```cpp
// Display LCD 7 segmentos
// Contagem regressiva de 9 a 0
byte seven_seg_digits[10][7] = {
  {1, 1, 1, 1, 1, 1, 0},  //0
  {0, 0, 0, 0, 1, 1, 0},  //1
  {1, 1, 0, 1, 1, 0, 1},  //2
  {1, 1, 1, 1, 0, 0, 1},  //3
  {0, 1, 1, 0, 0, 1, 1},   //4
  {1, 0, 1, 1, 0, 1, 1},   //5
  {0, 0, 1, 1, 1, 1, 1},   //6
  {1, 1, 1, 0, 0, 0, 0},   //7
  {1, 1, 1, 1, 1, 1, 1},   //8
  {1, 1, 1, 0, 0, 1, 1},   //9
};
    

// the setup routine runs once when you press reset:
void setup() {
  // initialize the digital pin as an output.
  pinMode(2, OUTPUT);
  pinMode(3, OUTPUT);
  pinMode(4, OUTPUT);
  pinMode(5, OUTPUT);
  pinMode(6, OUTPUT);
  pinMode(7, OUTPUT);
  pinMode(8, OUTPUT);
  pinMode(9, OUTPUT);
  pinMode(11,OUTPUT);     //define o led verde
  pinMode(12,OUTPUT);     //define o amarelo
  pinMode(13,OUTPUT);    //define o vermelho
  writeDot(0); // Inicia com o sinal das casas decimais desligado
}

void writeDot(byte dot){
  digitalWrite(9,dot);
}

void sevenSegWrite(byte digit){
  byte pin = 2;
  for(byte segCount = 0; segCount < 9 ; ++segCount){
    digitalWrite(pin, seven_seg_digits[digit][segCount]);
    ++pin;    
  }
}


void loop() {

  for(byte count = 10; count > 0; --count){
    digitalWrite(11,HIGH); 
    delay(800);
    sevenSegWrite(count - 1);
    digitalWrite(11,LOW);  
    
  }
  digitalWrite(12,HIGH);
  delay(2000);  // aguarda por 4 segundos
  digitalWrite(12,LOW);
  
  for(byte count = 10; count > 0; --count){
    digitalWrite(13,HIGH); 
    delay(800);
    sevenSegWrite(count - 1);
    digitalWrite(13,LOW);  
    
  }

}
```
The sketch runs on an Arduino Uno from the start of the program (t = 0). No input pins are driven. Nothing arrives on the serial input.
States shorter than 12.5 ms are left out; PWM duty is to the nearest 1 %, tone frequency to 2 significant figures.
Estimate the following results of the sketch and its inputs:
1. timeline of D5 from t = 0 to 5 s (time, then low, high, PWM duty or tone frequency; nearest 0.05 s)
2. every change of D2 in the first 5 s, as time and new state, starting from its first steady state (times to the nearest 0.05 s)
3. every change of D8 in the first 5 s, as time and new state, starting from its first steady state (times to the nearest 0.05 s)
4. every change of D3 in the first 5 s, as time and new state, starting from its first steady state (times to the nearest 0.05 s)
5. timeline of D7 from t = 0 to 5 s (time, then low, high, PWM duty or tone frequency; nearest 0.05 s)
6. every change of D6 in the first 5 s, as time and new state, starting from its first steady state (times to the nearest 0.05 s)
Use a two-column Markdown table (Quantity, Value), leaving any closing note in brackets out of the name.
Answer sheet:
| Quantity | Value |
|---|---|
| timeline of D5 from t = 0 to 5 s | 0 s low; 1.6 s high; 2.4 s low; 3.2 s high; 4.8 s low |
| every change of D2 in the first 5 s, as time and new state, starting from its first steady state | 0 s low; 0.8 s high; 3.2 s low; 4 s high; 4.8 s low |
| every change of D8 in the first 5 s, as time and new state, starting from its first steady state | 0 s low; 0.8 s high; 2.4 s low; 3.2 s high |
| every change of D3 in the first 5 s, as time and new state, starting from its first steady state | 0 s low; 0.8 s high; 3.2 s low; 4.8 s high |
| timeline of D7 from t = 0 to 5 s | 0 s low; 0.8 s high; 2.4 s low; 3.2 s high |
| every change of D6 in the first 5 s, as time and new state, starting from its first steady state | 0 s low; 1.6 s high; 2.4 s low; 3.2 s high; 4 s low |
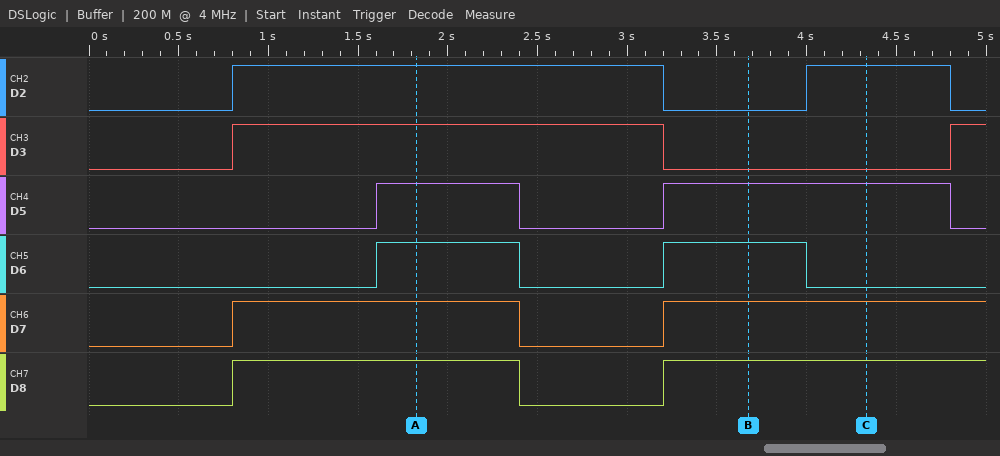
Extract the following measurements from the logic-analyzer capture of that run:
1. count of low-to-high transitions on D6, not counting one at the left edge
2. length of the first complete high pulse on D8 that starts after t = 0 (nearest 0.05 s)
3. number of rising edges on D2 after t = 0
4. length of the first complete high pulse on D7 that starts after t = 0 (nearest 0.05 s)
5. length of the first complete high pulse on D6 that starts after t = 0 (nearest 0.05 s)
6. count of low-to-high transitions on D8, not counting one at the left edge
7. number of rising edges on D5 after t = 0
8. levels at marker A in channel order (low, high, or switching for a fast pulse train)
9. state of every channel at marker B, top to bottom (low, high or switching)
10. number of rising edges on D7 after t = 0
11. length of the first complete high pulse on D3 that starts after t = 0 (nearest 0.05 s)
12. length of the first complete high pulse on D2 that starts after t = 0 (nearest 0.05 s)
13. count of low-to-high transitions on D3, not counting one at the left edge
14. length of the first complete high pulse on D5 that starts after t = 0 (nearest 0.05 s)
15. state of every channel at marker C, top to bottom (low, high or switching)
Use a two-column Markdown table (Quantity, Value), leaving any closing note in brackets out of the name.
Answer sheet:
| Quantity | Value |
|---|---|
| count of low-to-high transitions on D6, not counting one at the left edge | 2 |
| length of the first complete high pulse on D8 that starts after t = 0 | 1.60 s |
| number of rising edges on D2 after t = 0 | 2 |
| length of the first complete high pulse on D7 that starts after t = 0 | 1.60 s |
| length of the first complete high pulse on D6 that starts after t = 0 | 0.80 s |
| count of low-to-high transitions on D8, not counting one at the left edge | 2 |
| number of rising edges on D5 after t = 0 | 2 |
| levels at marker A in channel order | D2 high, D3 high, D5 high, D6 high, D7 high, D8 high |
| state of every channel at marker B, top to bottom | D2 low, D3 low, D5 high, D6 high, D7 high, D8 high |
| number of rising edges on D7 after t = 0 | 2 |
| length of the first complete high pulse on D3 that starts after t = 0 | 2.40 s |
| length of the first complete high pulse on D2 that starts after t = 0 | 2.40 s |
| count of low-to-high transitions on D3, not counting one at the left edge | 2 |
| length of the first complete high pulse on D5 that starts after t = 0 | 0.80 s |
| state of every channel at marker C, top to bottom | D2 high, D3 low, D5 high, D6 low, D7 high, D8 high |
